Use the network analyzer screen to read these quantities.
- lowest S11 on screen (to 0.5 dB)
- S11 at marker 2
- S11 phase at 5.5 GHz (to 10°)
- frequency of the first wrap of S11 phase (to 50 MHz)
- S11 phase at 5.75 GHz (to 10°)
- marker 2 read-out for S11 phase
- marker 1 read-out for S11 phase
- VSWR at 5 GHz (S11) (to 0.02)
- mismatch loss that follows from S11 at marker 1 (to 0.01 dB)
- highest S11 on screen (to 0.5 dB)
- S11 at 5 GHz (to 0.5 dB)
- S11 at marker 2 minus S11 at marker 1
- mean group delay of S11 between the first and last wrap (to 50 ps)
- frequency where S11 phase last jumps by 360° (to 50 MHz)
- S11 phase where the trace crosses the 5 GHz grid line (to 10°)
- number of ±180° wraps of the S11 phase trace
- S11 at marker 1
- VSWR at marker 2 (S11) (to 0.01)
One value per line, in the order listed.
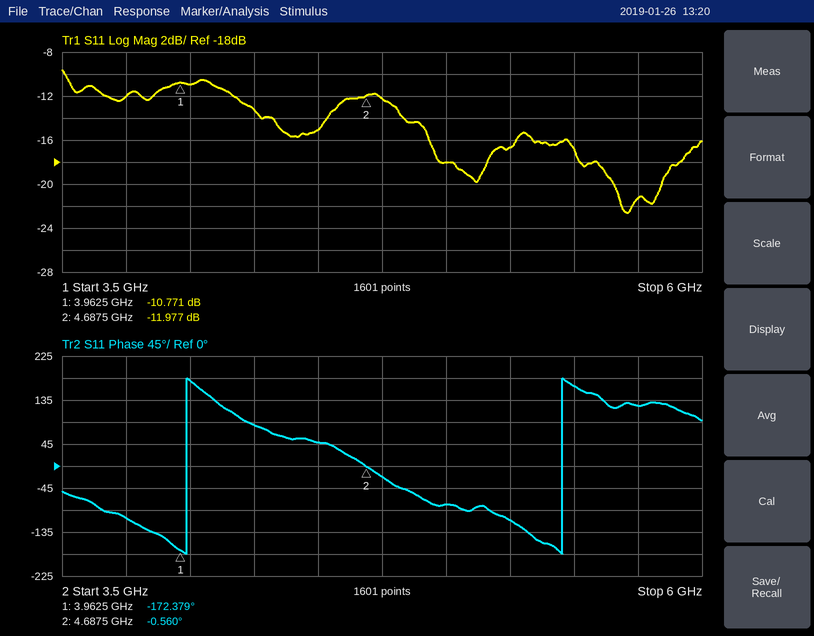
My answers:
-22.5 dB
-11.977 dB
160°
4.00 GHz
120°
-0.560°
-172.379°
1.28
0.38 dB
-9.5 dB
-18.0 dB
-1.206 dB
700 ps
5.45 GHz
-80°
2
-10.771 dB
1.67
